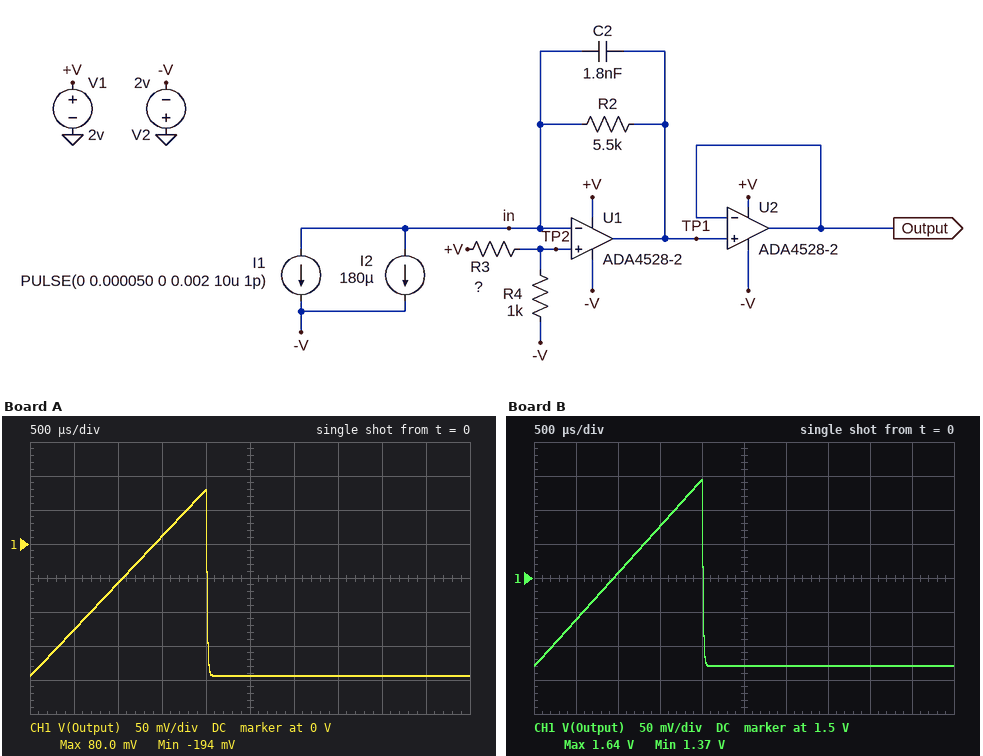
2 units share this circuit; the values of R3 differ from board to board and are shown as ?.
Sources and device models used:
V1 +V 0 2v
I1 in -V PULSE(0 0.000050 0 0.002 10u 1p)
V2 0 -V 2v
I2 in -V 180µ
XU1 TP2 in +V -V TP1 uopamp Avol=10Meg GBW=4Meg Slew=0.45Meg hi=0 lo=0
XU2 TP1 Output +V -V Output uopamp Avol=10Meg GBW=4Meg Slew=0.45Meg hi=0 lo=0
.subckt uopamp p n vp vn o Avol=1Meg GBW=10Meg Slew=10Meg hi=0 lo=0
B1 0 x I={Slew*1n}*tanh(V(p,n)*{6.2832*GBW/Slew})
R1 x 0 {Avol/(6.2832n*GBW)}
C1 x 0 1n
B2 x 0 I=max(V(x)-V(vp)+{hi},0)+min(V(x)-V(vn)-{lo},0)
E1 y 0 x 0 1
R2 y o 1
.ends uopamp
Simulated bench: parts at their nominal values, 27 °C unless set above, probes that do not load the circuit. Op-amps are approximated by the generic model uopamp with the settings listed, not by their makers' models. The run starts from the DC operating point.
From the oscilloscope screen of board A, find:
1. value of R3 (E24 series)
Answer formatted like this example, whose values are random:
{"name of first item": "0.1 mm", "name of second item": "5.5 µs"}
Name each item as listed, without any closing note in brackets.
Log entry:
{"value of R3": "3.9 kΩ"}
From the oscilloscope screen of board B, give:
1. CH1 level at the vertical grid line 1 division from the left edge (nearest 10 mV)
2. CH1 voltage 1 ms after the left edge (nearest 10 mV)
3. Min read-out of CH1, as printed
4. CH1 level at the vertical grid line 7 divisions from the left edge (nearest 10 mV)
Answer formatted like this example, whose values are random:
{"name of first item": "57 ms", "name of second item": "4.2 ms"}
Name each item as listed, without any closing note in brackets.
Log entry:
{"CH1 level at the vertical grid line 1 division from the left edge": "1.44 V", "CH1 voltage 1 ms after the left edge": "1.51 V", "Min read-out of CH1, as printed": "1.37 V", "CH1 level at the vertical grid line 7 divisions from the left edge": "1.37 V"}
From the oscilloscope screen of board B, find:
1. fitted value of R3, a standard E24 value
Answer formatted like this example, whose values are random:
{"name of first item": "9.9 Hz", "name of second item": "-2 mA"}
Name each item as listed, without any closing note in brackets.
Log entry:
{"fitted value of R3, a standard E24 value": "680 Ω"}
